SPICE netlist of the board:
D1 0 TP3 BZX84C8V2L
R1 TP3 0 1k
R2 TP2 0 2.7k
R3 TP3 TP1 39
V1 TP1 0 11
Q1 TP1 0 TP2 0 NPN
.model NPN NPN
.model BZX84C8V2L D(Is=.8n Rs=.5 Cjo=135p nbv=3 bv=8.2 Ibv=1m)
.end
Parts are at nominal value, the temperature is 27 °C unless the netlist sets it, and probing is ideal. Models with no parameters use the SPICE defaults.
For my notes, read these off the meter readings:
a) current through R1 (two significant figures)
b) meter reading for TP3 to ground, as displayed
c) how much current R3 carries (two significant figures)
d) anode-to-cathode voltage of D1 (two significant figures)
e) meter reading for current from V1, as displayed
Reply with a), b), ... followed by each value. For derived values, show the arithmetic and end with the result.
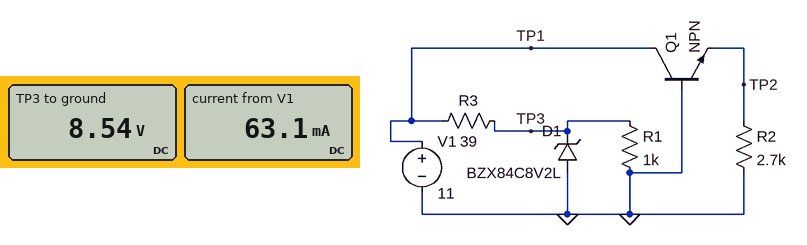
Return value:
a) (8.54 V) / 1 kΩ = 8.5 mA
b) 8.54 V
c) (11 V - 8.54 V) / 39 Ω = 63 mA
d) 0 V - 8.54 V = -8.5 V
e) 63.1 mA
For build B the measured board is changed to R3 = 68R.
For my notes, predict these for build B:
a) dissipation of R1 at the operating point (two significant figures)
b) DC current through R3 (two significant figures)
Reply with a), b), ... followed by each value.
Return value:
a) 72 mW
b) 37 mA
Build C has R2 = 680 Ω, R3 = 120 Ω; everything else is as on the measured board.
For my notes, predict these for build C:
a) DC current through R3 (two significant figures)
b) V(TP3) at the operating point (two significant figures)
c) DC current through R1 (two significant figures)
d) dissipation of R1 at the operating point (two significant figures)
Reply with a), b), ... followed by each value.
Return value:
a) 22 mA
b) 8.4 V
c) 8.4 mA
d) 71 mW
